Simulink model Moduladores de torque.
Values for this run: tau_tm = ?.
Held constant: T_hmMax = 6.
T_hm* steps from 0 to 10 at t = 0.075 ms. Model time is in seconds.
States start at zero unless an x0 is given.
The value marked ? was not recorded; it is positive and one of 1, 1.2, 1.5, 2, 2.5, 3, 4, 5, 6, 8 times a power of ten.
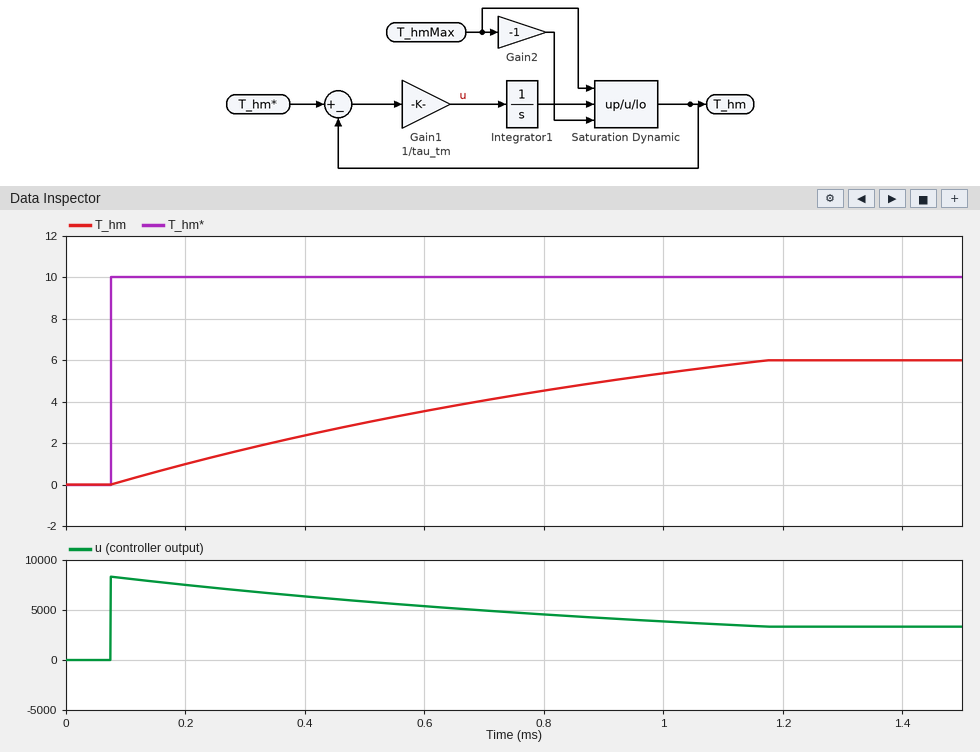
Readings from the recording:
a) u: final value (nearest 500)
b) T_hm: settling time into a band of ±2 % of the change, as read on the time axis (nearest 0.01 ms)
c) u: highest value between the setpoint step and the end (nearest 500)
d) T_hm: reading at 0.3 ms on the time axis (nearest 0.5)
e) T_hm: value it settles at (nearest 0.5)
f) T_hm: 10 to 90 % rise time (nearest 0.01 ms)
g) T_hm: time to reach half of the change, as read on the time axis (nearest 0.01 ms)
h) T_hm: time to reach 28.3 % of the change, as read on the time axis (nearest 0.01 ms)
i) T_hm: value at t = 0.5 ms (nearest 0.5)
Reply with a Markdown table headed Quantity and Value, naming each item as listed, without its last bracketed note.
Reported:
| Quantity | Value |
|---|---|
| u: final value | 3500 |
| T_hm: settling time into a band of ±2 % of the change, as read on the time axis | 1.14 ms |
| u: highest value between the setpoint step and the end | 8500 |
| T_hm: reading at 0.3 ms on the time axis | 1.5 |
| T_hm: value it settles at | 6.0 |
| T_hm: 10 to 90 % rise time | 0.86 ms |
| T_hm: time to reach half of the change, as read on the time axis | 0.50 ms |
| T_hm: time to reach 28.3 % of the change, as read on the time axis | 0.30 ms |
| T_hm: value at t = 0.5 ms | 3.0 |
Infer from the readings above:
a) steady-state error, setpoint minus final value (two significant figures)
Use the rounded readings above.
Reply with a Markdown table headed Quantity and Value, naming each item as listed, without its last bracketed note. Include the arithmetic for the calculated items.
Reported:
| Quantity | Value |
|---|---|
| steady-state error, setpoint minus final value | 10 - 6 = 4.0 |
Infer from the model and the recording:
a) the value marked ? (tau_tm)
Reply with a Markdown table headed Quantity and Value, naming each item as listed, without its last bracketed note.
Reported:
| Quantity | Value |
|---|---|
| the value marked ? | 0.0012 |
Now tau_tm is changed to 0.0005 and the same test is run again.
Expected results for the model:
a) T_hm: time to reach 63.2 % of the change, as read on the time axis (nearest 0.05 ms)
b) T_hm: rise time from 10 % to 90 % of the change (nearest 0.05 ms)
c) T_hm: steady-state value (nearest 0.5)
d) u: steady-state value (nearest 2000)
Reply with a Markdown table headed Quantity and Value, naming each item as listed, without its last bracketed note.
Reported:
| Quantity | Value |
|---|---|
| T_hm: time to reach 63.2 % of the change, as read on the time axis | 0.30 ms |
| T_hm: rise time from 10 % to 90 % of the change | 0.35 ms |
| T_hm: steady-state value | 6.0 |
| u: steady-state value | 8000 |
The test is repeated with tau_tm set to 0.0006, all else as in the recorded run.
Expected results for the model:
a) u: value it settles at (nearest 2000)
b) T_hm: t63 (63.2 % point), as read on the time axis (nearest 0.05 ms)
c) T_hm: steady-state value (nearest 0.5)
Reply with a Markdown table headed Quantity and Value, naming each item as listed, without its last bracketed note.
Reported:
| Quantity | Value |
|---|---|
| u: value it settles at | 6000 |
| T_hm: t63 (63.2 % point), as read on the time axis | 0.35 ms |
| T_hm: steady-state value | 6.0 |
